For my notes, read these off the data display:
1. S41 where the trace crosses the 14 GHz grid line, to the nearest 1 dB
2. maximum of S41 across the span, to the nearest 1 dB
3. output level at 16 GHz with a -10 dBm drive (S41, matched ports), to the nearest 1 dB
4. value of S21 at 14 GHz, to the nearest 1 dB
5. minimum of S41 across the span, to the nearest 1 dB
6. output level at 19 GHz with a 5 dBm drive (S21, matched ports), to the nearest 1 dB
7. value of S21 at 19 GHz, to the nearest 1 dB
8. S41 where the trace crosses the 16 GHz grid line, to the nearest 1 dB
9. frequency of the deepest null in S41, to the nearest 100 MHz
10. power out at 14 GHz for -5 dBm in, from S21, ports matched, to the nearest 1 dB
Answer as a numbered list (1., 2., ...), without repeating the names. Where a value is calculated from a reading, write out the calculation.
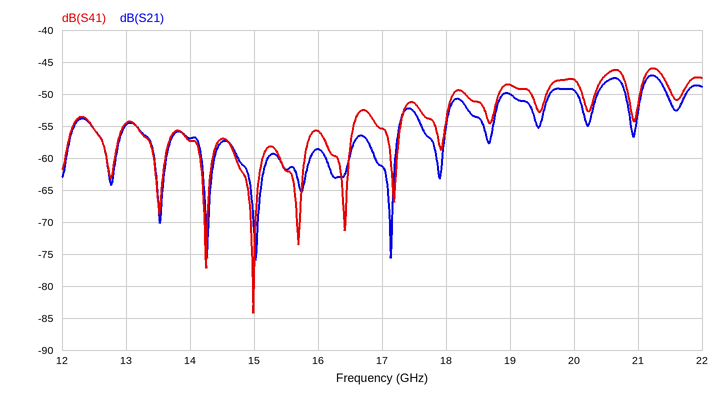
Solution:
1. -57 dB
2. -46 dB
3. -10 dBm + (-56 dB) = -66 dBm
4. -57 dB
5. -84 dB
6. 5 dBm + (-50 dB) = -45 dBm
7. -50 dB
8. -56 dB
9. 15.0 GHz
10. -5 dBm + (-57 dB) = -62 dBm
